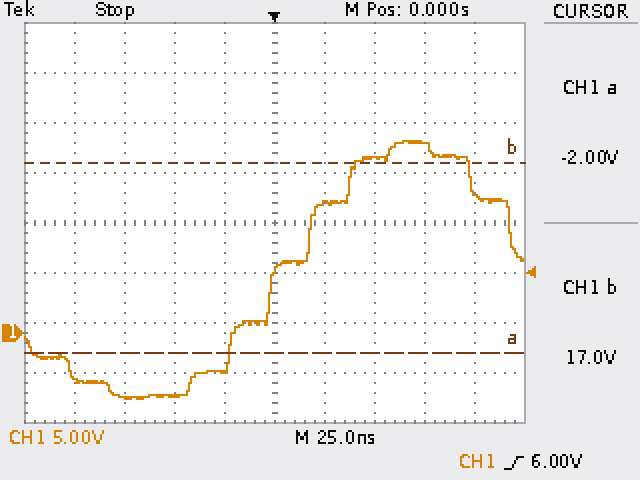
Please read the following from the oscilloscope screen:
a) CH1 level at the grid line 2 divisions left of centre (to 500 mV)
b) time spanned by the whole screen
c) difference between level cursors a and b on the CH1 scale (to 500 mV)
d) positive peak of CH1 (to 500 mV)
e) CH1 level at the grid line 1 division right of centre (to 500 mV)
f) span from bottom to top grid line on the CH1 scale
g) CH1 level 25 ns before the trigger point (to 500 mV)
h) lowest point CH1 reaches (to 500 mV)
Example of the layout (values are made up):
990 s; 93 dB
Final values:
-6.5 V; 250 ns; 19.0 V; 19.0 V; 13.0 V; 40 V; -3.5 V; -6.5 V
